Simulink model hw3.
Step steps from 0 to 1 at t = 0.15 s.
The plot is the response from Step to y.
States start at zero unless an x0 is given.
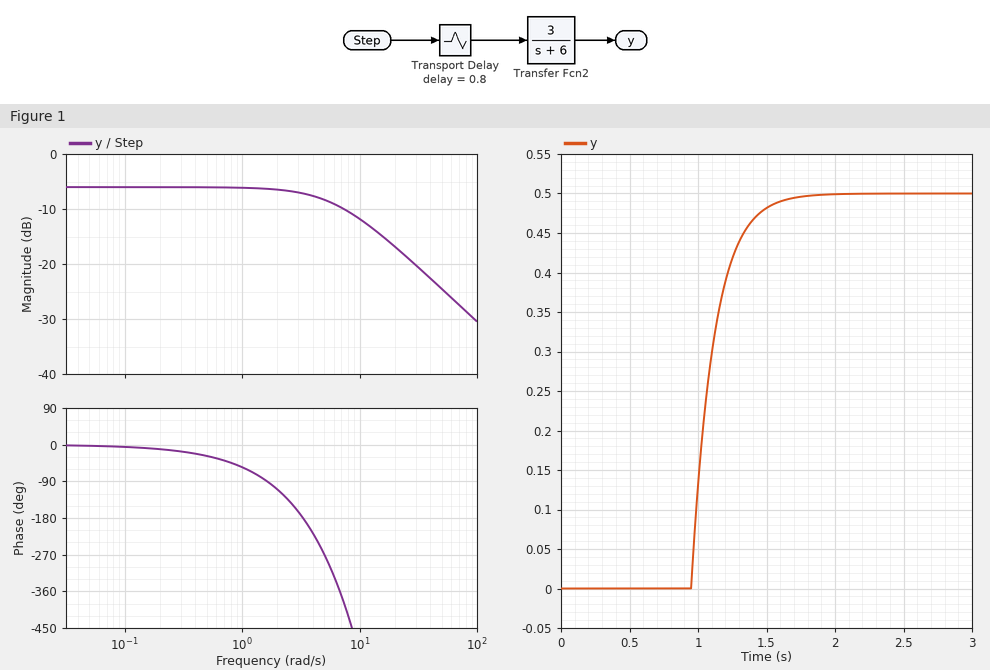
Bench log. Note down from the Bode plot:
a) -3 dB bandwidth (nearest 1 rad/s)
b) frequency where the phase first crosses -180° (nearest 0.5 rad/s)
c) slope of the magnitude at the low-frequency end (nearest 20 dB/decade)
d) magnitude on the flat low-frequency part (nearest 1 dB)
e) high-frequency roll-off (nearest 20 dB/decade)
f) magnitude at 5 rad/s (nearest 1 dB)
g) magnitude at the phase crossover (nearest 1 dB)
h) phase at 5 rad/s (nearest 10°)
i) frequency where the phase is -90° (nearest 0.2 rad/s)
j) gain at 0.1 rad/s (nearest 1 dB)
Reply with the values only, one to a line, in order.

6 rad/s
3.5 rad/s
0 dB/decade
-6 dB
-20 dB/decade
-8 dB
-7 dB
-270°
1.6 rad/s
-6 dB
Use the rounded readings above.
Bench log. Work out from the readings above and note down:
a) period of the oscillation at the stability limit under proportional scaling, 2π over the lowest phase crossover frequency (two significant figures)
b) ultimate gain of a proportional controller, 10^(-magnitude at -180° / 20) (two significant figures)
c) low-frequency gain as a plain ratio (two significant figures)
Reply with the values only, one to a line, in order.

1.8 s
2.2
0.50
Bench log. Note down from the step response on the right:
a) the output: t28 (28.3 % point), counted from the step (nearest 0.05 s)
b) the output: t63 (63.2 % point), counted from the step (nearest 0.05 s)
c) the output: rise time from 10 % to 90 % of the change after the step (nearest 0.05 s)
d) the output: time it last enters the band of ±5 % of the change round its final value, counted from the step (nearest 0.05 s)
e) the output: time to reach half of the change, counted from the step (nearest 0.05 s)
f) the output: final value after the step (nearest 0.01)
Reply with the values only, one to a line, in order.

0.85 s
0.95 s
0.35 s
1.30 s
0.90 s
0.50
